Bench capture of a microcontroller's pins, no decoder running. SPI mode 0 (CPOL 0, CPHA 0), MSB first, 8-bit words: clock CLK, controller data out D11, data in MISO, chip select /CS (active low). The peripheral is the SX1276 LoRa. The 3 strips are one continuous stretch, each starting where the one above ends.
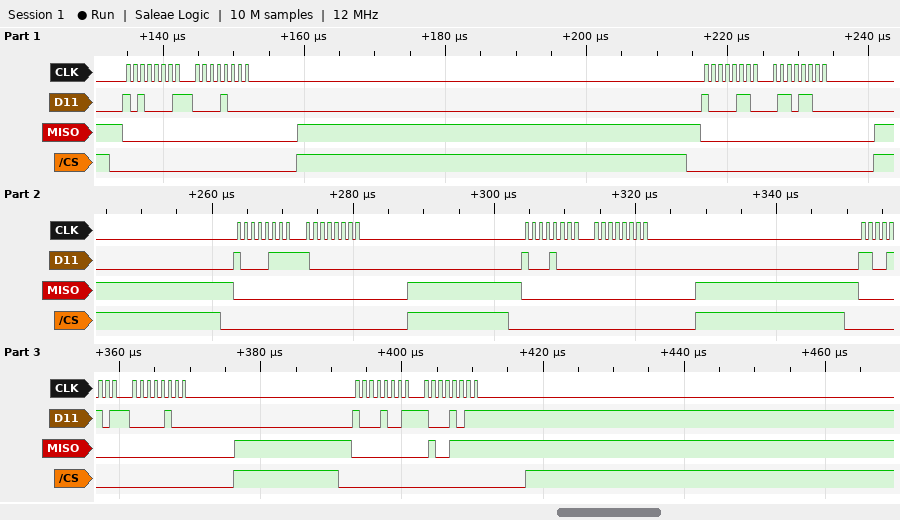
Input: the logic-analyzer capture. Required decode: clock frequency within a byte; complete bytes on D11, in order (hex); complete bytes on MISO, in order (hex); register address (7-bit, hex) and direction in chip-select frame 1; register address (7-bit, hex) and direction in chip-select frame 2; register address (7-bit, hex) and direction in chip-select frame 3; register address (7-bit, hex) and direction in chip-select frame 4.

1 MHz
0xA1 0x08 0x86 0x6C 0x87 0x80 0x88 0x00 0xCD 0x04 0x89 0x8B
0x00 0x00 0x00 0x00 0x00 0x00 0x00 0x00 0x00 0x00 0x00 0x4F
0x21 write
0x06 write
0x07 write
0x08 write
